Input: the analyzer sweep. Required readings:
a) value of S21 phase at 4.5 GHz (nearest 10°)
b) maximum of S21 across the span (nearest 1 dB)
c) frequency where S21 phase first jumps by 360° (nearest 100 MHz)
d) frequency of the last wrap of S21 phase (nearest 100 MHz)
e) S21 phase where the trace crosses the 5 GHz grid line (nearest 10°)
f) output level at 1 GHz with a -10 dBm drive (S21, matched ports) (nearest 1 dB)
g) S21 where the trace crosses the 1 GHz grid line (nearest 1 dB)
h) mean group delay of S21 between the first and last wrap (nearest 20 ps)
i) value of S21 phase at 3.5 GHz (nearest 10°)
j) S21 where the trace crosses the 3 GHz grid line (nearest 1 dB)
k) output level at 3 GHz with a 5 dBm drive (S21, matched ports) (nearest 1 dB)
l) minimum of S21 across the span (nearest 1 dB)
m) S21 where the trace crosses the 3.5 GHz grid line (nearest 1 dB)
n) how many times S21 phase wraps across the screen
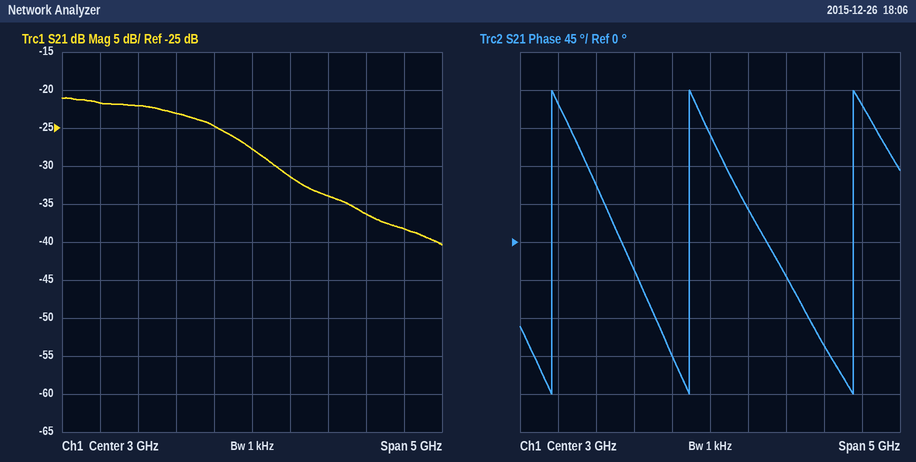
-120°
-21 dB
900 MHz
4.9 GHz
160°
-32 dBm
-22 dB
500 ps
40°
-28 dB
-23 dBm
-40 dB
-31 dB
3
